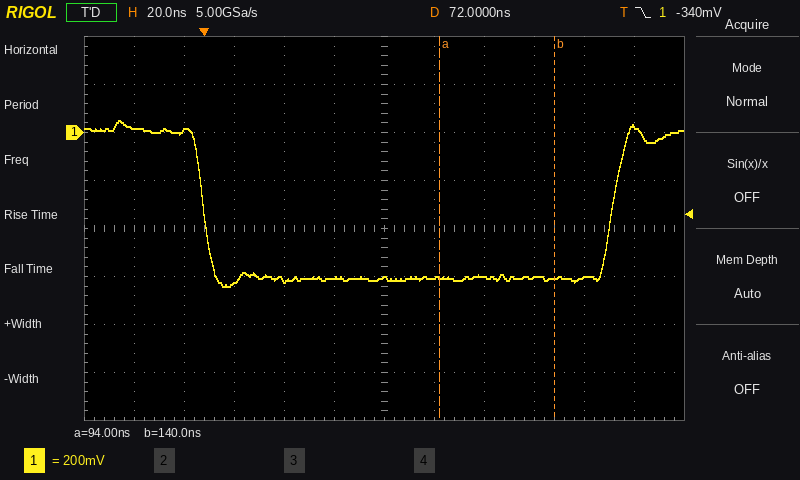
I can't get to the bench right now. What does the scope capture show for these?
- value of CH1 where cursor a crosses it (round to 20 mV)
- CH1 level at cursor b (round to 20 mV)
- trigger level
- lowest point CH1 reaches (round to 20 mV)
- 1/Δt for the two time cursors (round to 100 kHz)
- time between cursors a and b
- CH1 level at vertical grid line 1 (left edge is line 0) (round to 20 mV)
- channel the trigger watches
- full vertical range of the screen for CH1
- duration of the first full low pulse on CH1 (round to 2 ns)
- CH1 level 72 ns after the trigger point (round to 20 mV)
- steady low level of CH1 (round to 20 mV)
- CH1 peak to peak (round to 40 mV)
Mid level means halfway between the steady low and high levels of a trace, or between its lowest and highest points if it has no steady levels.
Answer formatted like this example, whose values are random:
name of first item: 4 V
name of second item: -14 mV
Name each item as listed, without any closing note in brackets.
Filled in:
value of CH1 where cursor a crosses it: -600 mV
CH1 level at cursor b: -600 mV
trigger level: -340 mV
lowest point CH1 reaches: -640 mV
1/Δt for the two time cursors: 21.7 MHz
time between cursors a and b: 46 ns
CH1 level at vertical grid line 1 (left edge is line 0): 20 mV
channel the trigger watches: CH1
full vertical range of the screen for CH1: 1.6 V
duration of the first full low pulse on CH1: 164 ns
CH1 level 72 ns after the trigger point: -600 mV
steady low level of CH1: -600 mV
CH1 peak to peak: 680 mV
